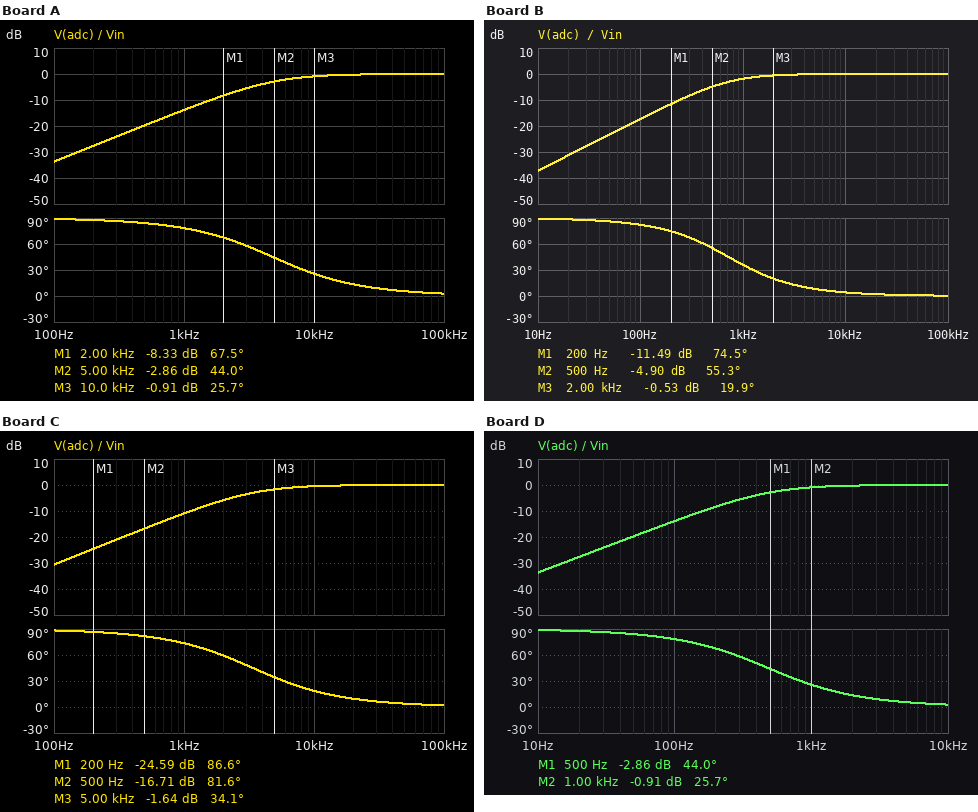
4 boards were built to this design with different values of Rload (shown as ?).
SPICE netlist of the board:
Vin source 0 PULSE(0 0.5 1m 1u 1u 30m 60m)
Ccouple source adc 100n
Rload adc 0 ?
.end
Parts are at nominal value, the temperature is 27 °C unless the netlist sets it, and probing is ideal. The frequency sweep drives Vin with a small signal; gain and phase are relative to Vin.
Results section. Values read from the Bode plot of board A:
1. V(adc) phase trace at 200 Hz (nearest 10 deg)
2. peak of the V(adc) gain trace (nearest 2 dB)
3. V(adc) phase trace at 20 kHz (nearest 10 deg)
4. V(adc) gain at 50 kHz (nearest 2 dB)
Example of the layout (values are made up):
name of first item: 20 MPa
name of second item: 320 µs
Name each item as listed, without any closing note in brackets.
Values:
V(adc) phase trace at 200 Hz: 90 deg
peak of the V(adc) gain trace: 0 dB
V(adc) phase trace at 20 kHz: 10 deg
V(adc) gain at 50 kHz: 0 dB
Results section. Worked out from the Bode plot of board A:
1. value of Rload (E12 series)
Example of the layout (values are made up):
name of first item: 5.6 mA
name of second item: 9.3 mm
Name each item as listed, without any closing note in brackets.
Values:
value of Rload: 330 Ω
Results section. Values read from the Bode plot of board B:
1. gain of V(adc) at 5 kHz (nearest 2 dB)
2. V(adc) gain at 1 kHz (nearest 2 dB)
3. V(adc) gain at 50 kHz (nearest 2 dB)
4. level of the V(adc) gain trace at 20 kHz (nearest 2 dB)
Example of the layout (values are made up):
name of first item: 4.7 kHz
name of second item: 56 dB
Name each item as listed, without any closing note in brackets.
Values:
gain of V(adc) at 5 kHz: 0 dB
V(adc) gain at 1 kHz: -2 dB
V(adc) gain at 50 kHz: 0 dB
level of the V(adc) gain trace at 20 kHz: 0 dB
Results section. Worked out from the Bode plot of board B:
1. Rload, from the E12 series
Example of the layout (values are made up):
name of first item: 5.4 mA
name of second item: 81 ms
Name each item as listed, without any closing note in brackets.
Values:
Rload, from the E12 series: 2.2 kΩ
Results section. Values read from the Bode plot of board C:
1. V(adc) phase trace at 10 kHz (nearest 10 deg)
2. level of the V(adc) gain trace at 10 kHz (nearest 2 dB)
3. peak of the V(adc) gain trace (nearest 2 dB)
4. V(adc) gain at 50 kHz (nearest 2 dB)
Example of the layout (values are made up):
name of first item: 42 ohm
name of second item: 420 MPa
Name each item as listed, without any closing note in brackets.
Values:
V(adc) phase trace at 10 kHz: 20 deg
level of the V(adc) gain trace at 10 kHz: 0 dB
peak of the V(adc) gain trace: 0 dB
V(adc) gain at 50 kHz: 0 dB
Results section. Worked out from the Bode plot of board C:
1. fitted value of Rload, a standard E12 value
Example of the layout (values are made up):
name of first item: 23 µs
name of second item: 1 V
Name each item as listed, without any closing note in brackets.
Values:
fitted value of Rload, a standard E12 value: 470 Ω
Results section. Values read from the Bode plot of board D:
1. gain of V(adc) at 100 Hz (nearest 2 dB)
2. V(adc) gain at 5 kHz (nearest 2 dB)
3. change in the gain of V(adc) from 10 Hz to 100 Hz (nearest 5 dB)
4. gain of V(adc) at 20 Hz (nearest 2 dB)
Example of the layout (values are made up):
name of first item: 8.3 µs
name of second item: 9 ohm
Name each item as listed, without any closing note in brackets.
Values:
gain of V(adc) at 100 Hz: -14 dB
V(adc) gain at 5 kHz: 0 dB
change in the gain of V(adc) from 10 Hz to 100 Hz: 20 dB
gain of V(adc) at 20 Hz: -28 dB
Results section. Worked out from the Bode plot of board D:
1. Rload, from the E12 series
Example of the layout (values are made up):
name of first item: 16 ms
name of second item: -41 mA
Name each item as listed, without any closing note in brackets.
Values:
Rload, from the E12 series: 3.3 kΩ
